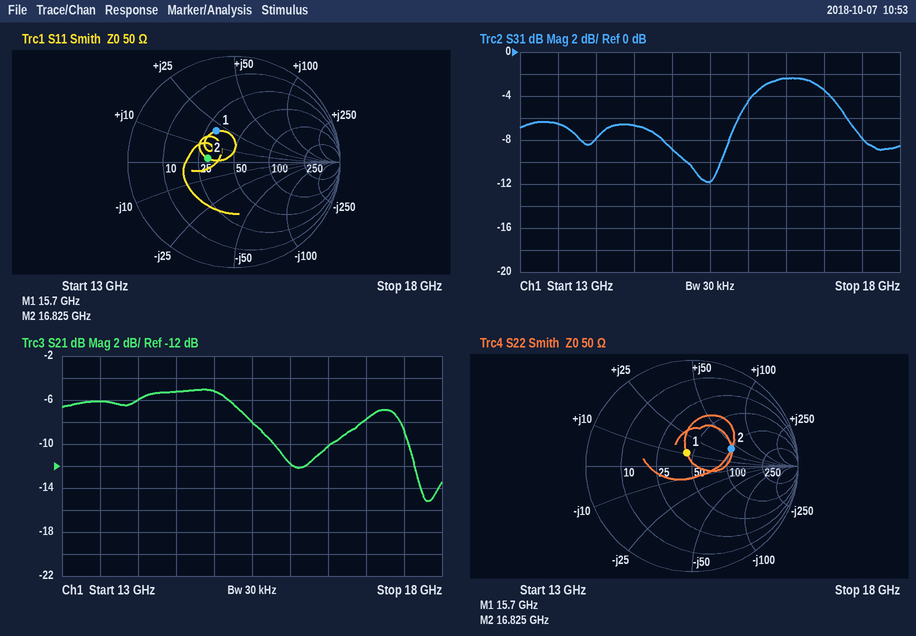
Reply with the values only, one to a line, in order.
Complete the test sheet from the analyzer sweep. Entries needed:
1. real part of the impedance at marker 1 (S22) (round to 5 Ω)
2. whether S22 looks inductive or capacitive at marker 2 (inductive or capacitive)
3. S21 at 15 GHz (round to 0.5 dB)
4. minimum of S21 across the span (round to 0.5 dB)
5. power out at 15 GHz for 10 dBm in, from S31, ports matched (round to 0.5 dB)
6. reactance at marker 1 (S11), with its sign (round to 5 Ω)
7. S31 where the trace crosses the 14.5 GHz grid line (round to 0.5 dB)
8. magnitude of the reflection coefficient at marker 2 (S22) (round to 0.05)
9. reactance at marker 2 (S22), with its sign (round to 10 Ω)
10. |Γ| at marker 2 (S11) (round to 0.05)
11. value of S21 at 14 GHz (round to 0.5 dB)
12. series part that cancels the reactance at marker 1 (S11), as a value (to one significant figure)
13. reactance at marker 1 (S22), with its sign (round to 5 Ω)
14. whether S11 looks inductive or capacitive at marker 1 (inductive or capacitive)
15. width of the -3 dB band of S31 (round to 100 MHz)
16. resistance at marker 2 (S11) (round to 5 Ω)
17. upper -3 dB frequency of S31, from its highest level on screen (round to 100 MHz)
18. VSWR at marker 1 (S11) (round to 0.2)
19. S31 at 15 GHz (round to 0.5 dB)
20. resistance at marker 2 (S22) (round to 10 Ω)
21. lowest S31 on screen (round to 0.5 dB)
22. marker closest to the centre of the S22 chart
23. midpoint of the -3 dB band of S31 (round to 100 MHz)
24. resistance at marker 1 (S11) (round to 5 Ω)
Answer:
45 Ω
inductive
-5.0 dB
-15.0 dB
1.0 dBm
+20 Ω
-6.5 dB
0.40
+40 Ω
0.25
-6.0 dB
500 fF
+10 Ω
inductive
1.3 GHz
30 Ω
17.2 GHz
2.0
-9.0 dB
100 Ω
-12.0 dB
marker 1
16.6 GHz
30 Ω
